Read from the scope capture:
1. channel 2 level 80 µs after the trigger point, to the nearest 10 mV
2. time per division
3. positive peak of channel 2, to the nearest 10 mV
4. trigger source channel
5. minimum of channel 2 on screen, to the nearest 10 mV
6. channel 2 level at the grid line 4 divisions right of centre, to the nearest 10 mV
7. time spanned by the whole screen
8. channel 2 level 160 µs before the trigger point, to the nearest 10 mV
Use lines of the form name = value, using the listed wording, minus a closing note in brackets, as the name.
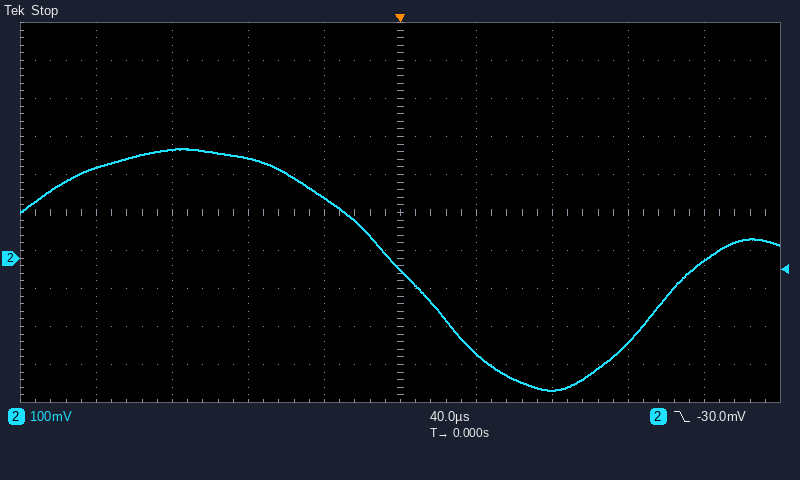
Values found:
channel 2 level 80 µs after the trigger point, to the nearest 10 mV = -350 mV
time per division = 40 µs
positive peak of channel 2, to the nearest 10 mV = 290 mV
trigger source channel = channel 2
minimum of channel 2 on screen, to the nearest 10 mV = -350 mV
channel 2 level at the grid line 4 divisions right of centre, to the nearest 10 mV = -10 mV
time spanned by the whole screen = 400 µs
channel 2 level 160 µs before the trigger point, to the nearest 10 mV = 240 mV
